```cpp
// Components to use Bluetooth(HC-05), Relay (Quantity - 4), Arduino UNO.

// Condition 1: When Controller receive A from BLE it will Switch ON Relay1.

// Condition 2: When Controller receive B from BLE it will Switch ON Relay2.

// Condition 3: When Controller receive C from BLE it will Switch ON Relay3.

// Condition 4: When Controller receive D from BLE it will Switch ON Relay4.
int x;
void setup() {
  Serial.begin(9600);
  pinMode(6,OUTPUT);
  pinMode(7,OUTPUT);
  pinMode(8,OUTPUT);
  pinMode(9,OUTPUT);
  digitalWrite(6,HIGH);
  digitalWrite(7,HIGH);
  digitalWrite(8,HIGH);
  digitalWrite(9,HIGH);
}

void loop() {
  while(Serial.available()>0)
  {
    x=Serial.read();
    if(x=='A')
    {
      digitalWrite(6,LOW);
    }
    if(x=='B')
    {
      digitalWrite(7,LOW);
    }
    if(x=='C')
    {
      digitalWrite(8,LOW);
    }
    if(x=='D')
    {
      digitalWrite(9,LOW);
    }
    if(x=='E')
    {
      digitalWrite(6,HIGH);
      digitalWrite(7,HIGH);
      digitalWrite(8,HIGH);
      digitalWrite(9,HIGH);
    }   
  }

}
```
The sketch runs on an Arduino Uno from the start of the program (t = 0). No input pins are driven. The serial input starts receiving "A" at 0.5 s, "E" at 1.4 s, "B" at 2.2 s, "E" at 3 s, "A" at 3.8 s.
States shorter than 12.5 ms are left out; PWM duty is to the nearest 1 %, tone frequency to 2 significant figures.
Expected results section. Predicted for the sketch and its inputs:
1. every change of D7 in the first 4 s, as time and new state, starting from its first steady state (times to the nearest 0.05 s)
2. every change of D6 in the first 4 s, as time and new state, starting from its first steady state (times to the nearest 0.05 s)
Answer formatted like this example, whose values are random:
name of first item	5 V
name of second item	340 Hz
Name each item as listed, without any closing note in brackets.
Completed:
every change of D7 in the first 4 s, as time and new state, starting from its first steady state	0 s high; 2.2 s low; 3 s high
every change of D6 in the first 4 s, as time and new state, starting from its first steady state	0 s high; 0.5 s low; 1.4 s high; 3.8 s low
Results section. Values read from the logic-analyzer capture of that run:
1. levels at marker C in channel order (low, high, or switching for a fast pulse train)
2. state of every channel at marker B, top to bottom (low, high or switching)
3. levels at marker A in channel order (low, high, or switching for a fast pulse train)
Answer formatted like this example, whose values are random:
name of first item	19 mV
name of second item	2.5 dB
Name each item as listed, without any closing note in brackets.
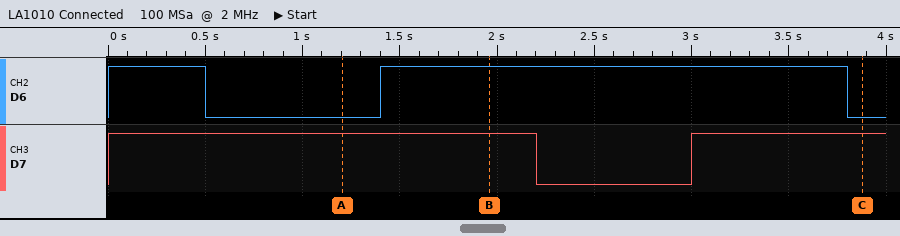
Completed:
levels at marker C in channel order	D6 low, D7 high
state of every channel at marker B, top to bottom	D6 high, D7 high
levels at marker A in channel order	D6 low, D7 high
